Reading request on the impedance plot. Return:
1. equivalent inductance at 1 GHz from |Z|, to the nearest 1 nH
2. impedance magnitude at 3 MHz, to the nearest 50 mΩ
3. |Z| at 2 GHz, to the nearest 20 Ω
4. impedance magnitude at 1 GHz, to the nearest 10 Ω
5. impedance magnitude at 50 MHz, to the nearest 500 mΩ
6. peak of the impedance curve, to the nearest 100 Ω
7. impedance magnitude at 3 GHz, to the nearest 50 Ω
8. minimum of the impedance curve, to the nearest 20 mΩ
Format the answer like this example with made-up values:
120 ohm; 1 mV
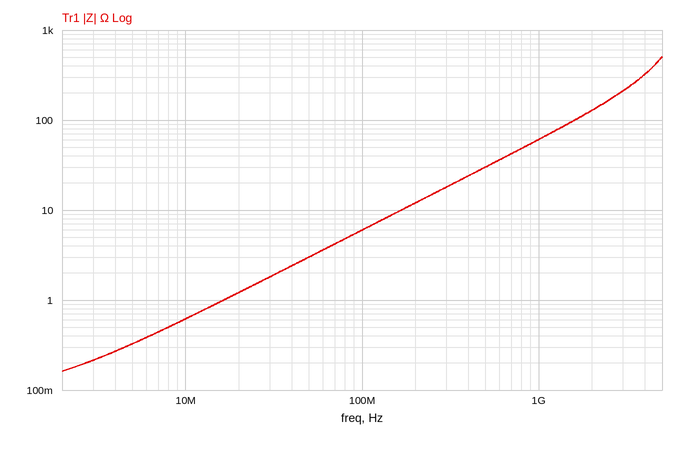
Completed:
10 nH; 200 mΩ; 120 Ω; 60 Ω; 3.0 Ω; 500 Ω; 200 Ω; 160 mΩ
